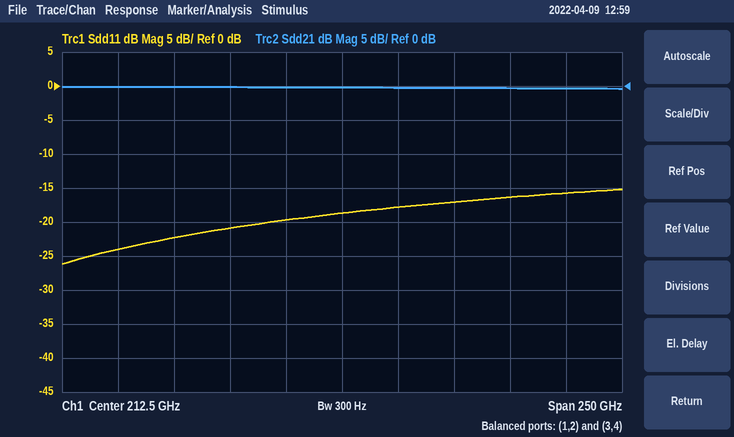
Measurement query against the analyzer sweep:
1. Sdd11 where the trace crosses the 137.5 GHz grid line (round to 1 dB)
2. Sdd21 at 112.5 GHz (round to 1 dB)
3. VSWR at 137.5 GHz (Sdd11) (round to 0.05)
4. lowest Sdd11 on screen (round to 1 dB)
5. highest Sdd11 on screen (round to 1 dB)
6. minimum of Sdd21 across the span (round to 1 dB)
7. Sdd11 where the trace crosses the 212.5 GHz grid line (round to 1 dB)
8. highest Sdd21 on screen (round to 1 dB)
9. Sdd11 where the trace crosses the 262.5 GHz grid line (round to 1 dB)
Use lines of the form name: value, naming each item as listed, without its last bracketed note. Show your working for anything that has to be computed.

Sdd11 where the trace crosses the 137.5 GHz grid line: -22 dB
Sdd21 at 112.5 GHz: 0 dB
VSWR at 137.5 GHz (Sdd11): |Γ| = 10^(-22/20) = 0.0794; VSWR = (1 + 0.0794)/(1 − 0.0794) ≈ 1.17, so 1.15 to the nearest 0.05
lowest Sdd11 on screen: -26 dB
highest Sdd11 on screen: -15 dB
minimum of Sdd21 across the span: 0 dB
Sdd11 where the trace crosses the 212.5 GHz grid line: -19 dB
highest Sdd21 on screen: 0 dB
Sdd11 where the trace crosses the 262.5 GHz grid line: -17 dB
